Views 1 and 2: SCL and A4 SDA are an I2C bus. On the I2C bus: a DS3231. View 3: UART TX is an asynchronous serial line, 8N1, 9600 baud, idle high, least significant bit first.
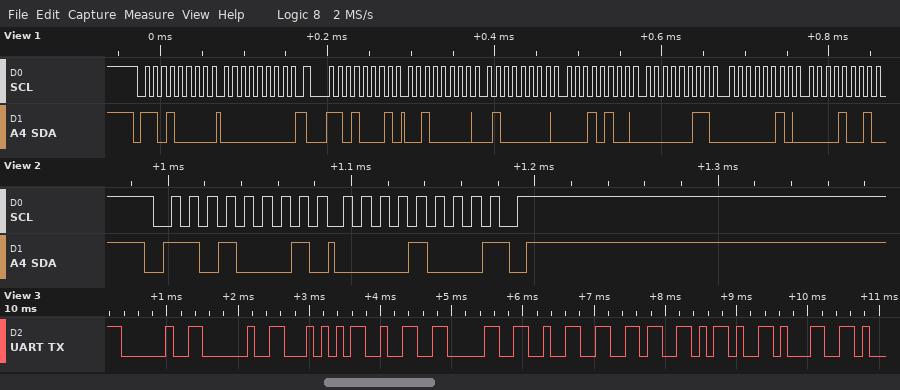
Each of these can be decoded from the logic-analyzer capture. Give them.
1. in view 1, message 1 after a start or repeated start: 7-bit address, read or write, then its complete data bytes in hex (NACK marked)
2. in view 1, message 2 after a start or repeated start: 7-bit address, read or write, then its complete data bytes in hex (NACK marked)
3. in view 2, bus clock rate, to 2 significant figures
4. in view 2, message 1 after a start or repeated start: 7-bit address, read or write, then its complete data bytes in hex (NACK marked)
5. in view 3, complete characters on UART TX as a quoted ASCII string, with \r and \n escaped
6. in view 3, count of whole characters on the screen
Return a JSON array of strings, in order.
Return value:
["0x68 write: 00", "0x68 read: 20 40 14 03 02 09", "100 kHz", "0x68 read: 08 NACK", "\"  T2026-1\"", "9"]
